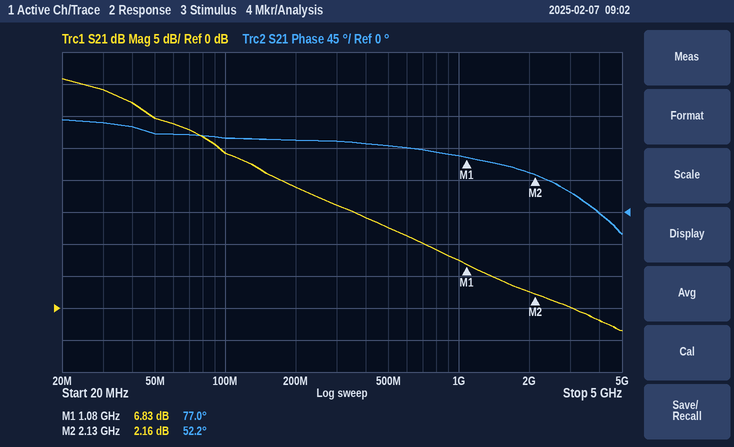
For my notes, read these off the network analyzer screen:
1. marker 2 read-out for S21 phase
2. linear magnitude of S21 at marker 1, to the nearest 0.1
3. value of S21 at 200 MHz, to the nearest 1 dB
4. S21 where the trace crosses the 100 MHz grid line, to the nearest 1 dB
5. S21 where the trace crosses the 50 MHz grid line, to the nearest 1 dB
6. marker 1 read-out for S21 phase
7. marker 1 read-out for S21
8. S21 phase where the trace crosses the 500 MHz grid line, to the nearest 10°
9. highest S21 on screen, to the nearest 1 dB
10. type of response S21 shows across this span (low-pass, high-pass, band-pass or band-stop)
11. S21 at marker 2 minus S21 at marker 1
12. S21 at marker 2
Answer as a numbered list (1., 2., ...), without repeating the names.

1. 52.2°
2. 2.2
3. 19 dB
4. 24 dB
5. 30 dB
6. 77.0°
7. 6.83 dB
8. 90°
9. 36 dB
10. low-pass
11. -4.67 dB
12. 2.16 dB
